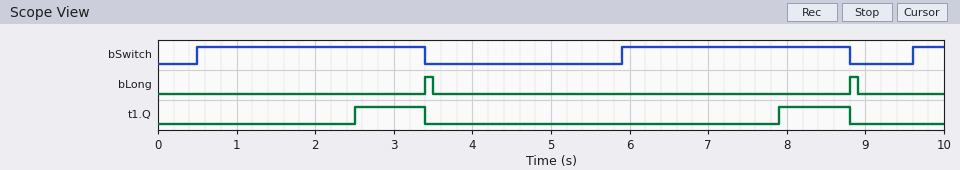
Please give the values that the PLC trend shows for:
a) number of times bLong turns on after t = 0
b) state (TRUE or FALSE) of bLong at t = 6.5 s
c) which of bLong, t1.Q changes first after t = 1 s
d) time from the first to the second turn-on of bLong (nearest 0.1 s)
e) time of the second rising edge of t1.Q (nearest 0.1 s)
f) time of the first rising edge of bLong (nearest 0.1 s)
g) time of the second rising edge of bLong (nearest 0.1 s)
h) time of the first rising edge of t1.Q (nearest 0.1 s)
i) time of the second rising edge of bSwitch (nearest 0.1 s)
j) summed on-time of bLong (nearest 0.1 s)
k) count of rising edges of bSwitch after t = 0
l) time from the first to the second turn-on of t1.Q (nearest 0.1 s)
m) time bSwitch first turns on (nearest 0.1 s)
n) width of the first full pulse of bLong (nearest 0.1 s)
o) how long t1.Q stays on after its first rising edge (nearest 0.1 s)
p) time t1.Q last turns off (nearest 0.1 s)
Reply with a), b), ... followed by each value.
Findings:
a) 2
b) FALSE
c) t1.Q
d) 5.4 s
e) 7.9 s
f) 3.4 s
g) 8.8 s
h) 2.5 s
i) 5.9 s
j) 0.2 s
k) 3
l) 5.4 s
m) 0.5 s
n) 0.1 s
o) 0.9 s
p) 8.8 s
